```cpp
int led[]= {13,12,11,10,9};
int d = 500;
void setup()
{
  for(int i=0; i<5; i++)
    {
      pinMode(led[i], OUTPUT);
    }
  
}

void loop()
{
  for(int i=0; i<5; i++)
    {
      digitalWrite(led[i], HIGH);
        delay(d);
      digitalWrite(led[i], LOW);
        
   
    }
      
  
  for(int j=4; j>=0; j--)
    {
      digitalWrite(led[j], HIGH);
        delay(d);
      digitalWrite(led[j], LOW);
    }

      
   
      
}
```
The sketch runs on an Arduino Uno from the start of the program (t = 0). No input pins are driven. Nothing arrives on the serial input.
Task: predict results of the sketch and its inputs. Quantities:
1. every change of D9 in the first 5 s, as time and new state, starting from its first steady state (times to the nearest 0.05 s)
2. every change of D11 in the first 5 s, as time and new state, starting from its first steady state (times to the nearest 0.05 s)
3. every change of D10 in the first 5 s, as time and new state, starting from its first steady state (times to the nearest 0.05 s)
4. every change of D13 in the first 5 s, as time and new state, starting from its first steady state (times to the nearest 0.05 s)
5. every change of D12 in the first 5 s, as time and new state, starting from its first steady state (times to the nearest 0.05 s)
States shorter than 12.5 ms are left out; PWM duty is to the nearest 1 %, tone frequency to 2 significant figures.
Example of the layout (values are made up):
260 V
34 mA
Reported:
0 s low; 2 s high; 3 s low
0 s low; 1 s high; 1.5 s low; 3.5 s high; 4 s low
0 s low; 1.5 s high; 2 s low; 3 s high; 3.5 s low
0 s high; 0.5 s low; 4.5 s high
0 s low; 0.5 s high; 1 s low; 4 s high; 4.5 s low
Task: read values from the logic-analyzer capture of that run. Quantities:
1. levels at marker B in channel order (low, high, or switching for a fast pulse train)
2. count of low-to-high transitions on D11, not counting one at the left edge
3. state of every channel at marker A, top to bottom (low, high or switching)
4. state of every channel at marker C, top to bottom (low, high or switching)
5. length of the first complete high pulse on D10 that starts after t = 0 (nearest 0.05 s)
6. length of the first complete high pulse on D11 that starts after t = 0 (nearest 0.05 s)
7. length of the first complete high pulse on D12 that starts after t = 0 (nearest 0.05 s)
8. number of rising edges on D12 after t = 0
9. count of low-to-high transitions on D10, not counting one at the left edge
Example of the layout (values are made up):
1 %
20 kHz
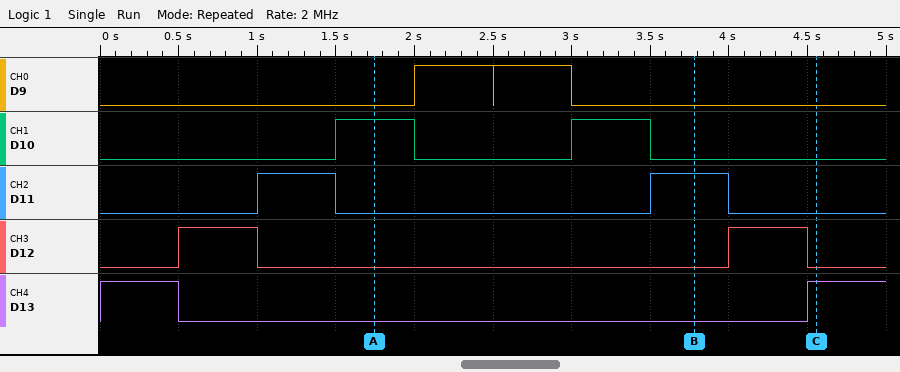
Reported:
D9 low, D10 low, D11 high, D12 low, D13 low
2
D9 low, D10 high, D11 low, D12 low, D13 low
D9 low, D10 low, D11 low, D12 low, D13 high
0.50 s
0.50 s
0.50 s
2
2
